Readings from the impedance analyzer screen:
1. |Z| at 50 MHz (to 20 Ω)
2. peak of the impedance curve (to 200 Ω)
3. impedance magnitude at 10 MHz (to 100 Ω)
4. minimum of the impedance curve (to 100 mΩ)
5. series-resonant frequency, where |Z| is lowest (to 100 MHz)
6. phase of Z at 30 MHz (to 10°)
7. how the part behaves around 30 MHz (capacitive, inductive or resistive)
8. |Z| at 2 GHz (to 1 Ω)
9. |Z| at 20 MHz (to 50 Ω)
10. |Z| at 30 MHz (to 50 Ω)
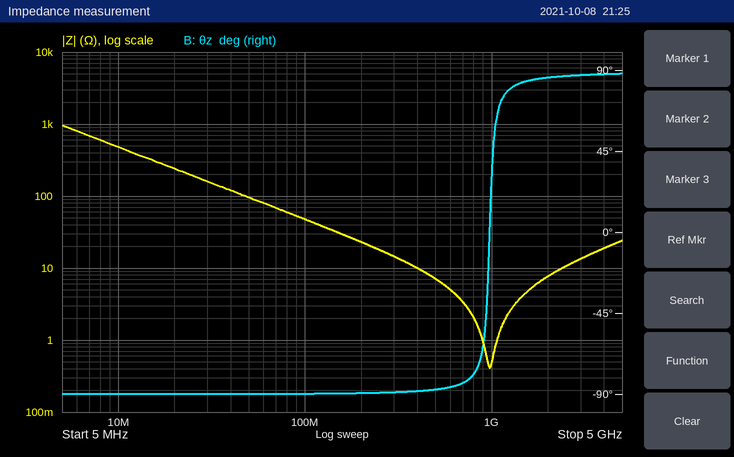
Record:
100 Ω
1.0 kΩ
500 Ω
400 mΩ
1.0 GHz
-90°
capacitive
8 Ω
250 Ω
150 Ω
